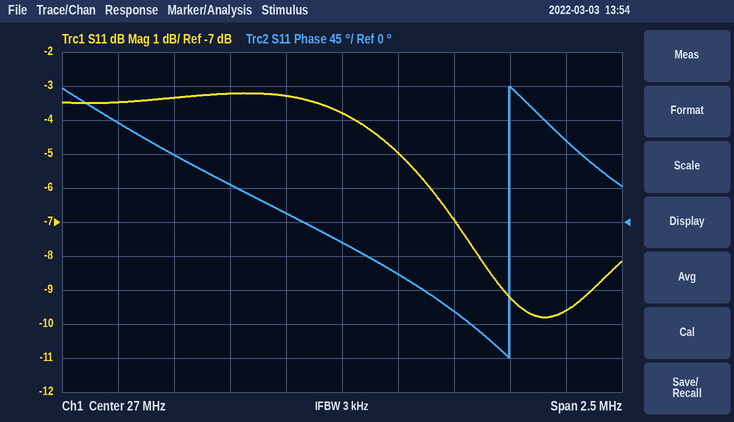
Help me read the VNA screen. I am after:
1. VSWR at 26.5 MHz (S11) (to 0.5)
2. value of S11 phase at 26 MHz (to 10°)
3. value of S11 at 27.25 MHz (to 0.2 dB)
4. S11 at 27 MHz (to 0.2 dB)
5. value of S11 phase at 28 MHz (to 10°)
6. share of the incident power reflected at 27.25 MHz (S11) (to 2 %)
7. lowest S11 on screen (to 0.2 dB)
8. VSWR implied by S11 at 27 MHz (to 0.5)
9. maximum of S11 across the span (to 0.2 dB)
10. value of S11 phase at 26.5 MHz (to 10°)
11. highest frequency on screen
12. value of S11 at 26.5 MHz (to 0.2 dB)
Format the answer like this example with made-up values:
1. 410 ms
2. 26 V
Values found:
1. 5.5
2. 130°
3. -5.0 dB
4. -3.8 dB
5. 110°
6. 32 %
7. -9.8 dB
8. 4.5
9. -3.2 dB
10. 50°
11. 28.25 MHz
12. -3.2 dB
